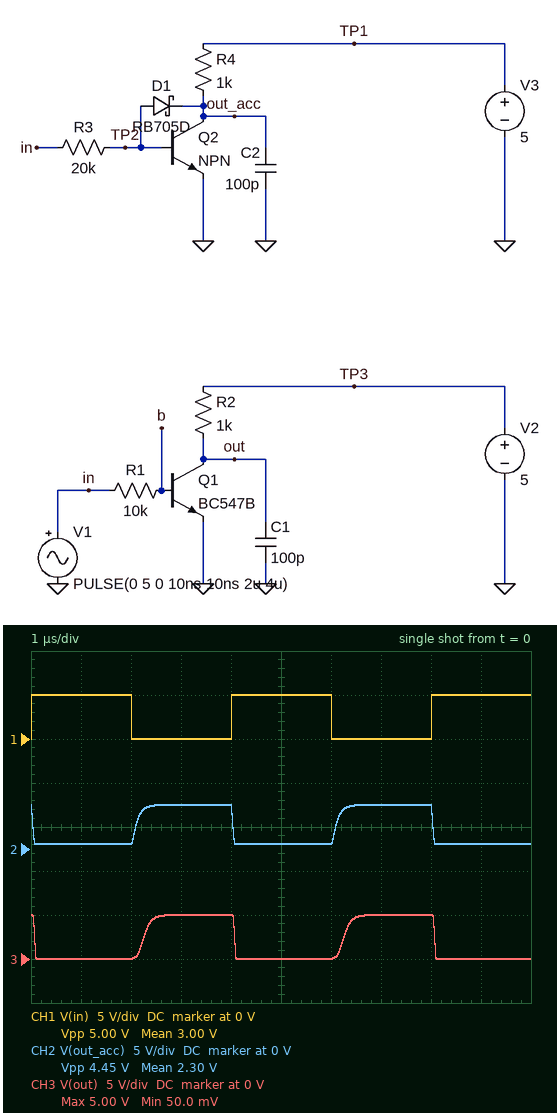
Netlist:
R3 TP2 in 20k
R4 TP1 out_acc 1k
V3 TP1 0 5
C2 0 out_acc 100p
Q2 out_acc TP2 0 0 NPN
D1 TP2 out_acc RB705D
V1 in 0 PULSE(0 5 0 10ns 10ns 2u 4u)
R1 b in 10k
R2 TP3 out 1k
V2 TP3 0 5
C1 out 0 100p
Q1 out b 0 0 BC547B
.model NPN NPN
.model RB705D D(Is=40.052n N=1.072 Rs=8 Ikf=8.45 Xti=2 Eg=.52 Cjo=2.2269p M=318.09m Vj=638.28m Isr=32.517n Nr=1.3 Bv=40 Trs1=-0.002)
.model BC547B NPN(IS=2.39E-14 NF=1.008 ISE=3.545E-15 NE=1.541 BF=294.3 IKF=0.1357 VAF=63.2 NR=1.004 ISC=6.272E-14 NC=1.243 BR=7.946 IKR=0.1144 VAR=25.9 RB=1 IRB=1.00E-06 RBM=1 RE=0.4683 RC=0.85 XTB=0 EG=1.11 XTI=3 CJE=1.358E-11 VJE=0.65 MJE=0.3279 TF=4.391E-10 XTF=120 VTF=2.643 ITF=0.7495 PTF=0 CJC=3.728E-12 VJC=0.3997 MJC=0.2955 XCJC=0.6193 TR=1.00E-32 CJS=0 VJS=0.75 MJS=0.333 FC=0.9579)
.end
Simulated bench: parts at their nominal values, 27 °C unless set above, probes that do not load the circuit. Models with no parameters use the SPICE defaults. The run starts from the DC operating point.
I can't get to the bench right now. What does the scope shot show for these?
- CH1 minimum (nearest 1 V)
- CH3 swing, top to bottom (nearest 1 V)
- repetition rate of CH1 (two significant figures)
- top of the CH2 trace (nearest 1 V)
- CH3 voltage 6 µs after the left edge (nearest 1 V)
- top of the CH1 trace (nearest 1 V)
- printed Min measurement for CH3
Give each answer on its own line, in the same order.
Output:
0 V
5 V
250 kHz
5 V
0 V
5 V
50.0 mV
